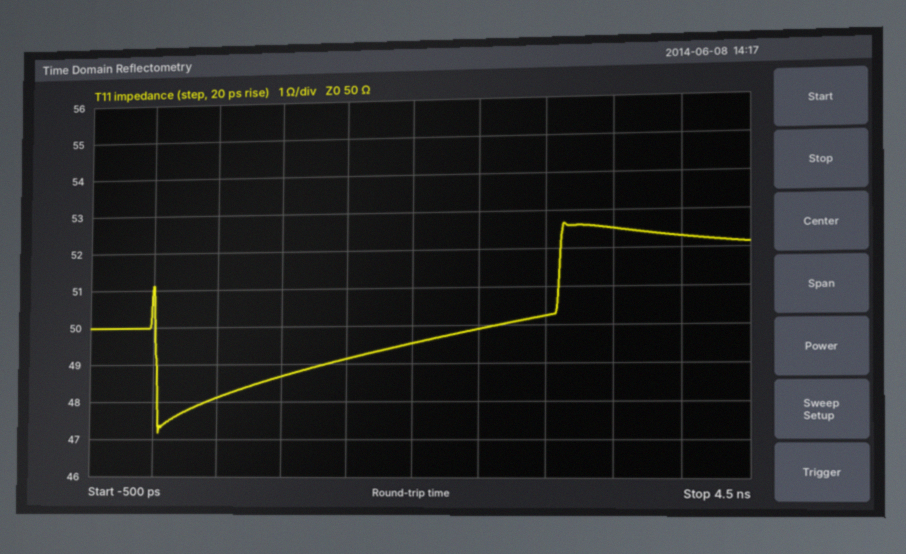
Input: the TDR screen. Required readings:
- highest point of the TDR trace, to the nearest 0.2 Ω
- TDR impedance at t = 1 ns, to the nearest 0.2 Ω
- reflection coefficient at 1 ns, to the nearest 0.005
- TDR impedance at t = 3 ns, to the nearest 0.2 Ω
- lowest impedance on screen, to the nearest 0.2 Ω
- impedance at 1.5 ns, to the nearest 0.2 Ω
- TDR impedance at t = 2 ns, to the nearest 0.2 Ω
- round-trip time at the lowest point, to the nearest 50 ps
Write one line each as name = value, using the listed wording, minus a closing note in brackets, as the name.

highest point of the TDR trace, to the nearest 0.2 Ω = 52.6 Ω
TDR impedance at t = 1 ns, to the nearest 0.2 Ω = 48.6 Ω
reflection coefficient at 1 ns, to the nearest 0.005 = -0.015
TDR impedance at t = 3 ns, to the nearest 0.2 Ω = 50.2 Ω
lowest impedance on screen, to the nearest 0.2 Ω = 47.2 Ω
impedance at 1.5 ns, to the nearest 0.2 Ω = 49.2 Ω
TDR impedance at t = 2 ns, to the nearest 0.2 Ω = 49.6 Ω
round-trip time at the lowest point, to the nearest 50 ps = 50 ps
